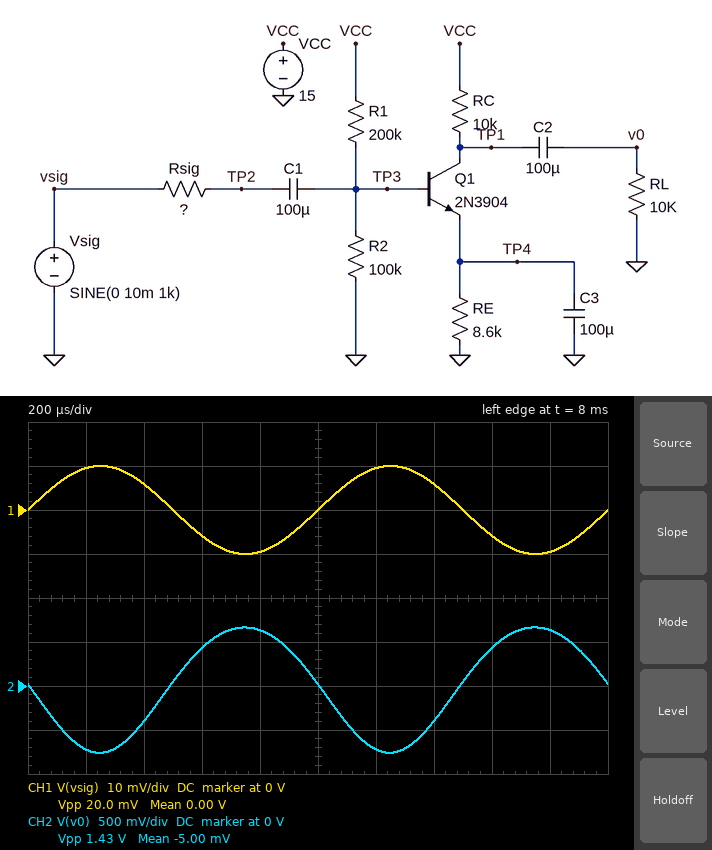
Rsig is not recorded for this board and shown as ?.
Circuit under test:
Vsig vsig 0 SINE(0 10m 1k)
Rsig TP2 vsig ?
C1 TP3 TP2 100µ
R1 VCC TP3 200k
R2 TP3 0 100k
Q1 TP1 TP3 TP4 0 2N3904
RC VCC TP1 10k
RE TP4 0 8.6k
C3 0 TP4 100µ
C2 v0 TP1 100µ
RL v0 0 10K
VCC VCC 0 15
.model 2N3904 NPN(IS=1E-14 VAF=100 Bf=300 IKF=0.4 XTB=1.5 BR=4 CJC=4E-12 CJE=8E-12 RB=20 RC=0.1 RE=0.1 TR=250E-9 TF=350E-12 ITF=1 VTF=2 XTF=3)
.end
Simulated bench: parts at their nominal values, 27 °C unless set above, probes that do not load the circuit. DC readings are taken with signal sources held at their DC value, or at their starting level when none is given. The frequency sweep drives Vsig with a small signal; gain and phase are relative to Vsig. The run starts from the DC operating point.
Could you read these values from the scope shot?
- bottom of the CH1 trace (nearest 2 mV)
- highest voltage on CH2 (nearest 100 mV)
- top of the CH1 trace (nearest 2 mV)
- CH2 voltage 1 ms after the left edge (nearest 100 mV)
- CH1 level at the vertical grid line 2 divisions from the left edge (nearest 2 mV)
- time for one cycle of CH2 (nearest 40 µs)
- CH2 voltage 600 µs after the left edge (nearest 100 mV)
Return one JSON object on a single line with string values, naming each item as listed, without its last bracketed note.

{"bottom of the CH1 trace": "-10 mV", "highest voltage on CH2": "700 mV", "top of the CH1 trace": "10 mV", "CH2 voltage 1 ms after the left edge": "0 V", "CH1 level at the vertical grid line 2 divisions from the left edge": "6 mV", "time for one cycle of CH2": "1.00 ms", "CH2 voltage 600 µs after the left edge": "400 mV"}
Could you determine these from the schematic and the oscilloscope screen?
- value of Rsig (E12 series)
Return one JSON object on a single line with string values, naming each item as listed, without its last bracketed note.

{"value of Rsig": "3.9 kΩ"}
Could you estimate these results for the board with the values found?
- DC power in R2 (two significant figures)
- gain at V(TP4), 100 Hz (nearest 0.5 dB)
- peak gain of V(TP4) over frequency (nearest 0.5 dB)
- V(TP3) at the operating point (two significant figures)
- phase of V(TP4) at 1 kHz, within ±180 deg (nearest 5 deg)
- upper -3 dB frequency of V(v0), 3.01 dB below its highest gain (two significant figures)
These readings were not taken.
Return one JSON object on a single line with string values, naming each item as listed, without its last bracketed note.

{"DC power in R2": "240 µW", "gain at V(TP4), 100 Hz": "-13.0 dB", "peak gain of V(TP4) over frequency": "-0.5 dB", "V(TP3) at the operating point": "4.9 V", "phase of V(TP4) at 1 kHz, within ±180 deg": "-90 deg", "upper -3 dB frequency of V(v0), 3.01 dB below its highest gain": "250 kHz"}
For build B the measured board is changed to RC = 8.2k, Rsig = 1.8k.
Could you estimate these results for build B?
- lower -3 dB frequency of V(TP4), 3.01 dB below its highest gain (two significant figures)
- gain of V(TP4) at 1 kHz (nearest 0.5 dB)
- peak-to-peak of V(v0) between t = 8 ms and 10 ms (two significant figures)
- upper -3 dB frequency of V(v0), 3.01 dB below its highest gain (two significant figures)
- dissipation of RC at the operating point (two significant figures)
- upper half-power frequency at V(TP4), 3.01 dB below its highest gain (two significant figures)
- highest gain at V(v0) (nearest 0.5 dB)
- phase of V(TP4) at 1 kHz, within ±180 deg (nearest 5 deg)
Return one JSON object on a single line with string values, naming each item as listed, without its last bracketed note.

{"lower -3 dB frequency of V(TP4), 3.01 dB below its highest gain": "24 mHz", "gain of V(TP4) at 1 kHz": "-31.5 dB", "peak-to-peak of V(v0) between t = 8 ms and 10 ms": "1.5 V", "upper -3 dB frequency of V(v0), 3.01 dB below its highest gain": "530 kHz", "dissipation of RC at the operating point": "2.0 mW", "upper half-power frequency at V(TP4), 3.01 dB below its highest gain": "27 Hz", "highest gain at V(v0)": "37.5 dB", "phase of V(TP4) at 1 kHz, within ±180 deg": "-90 deg"}
